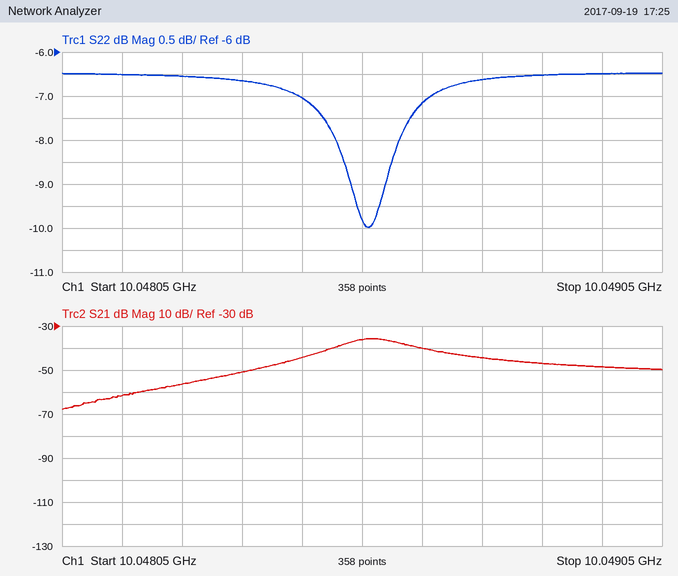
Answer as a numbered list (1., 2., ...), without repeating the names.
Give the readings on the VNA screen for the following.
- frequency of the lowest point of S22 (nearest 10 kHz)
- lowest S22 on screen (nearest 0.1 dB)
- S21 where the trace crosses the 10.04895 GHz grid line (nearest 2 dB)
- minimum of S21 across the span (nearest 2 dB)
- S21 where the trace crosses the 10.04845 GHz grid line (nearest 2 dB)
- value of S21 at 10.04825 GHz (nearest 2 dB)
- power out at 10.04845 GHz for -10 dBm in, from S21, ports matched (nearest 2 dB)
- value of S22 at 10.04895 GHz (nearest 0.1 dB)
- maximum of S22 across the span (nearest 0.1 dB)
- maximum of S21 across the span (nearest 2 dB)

1. 10.04856 GHz
2. -10.0 dB
3. -48 dB
4. -68 dB
5. -44 dB
6. -56 dB
7. -54 dBm
8. -6.5 dB
9. -6.5 dB
10. -36 dB
